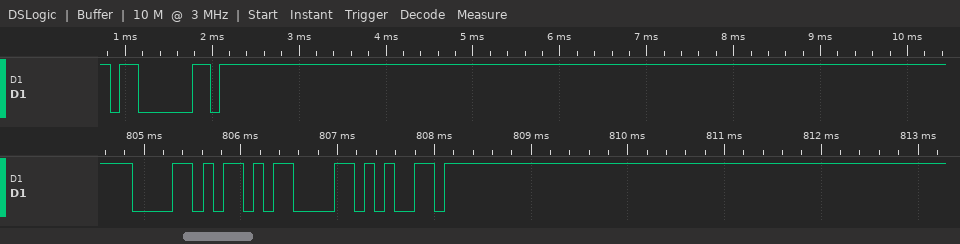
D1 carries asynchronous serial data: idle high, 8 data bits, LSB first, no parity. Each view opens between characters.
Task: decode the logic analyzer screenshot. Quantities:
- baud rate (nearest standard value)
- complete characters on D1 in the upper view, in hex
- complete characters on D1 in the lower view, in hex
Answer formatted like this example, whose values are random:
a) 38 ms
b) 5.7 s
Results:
a) 9600 baud
b) 03, FF
c) 58, 0D, 65
